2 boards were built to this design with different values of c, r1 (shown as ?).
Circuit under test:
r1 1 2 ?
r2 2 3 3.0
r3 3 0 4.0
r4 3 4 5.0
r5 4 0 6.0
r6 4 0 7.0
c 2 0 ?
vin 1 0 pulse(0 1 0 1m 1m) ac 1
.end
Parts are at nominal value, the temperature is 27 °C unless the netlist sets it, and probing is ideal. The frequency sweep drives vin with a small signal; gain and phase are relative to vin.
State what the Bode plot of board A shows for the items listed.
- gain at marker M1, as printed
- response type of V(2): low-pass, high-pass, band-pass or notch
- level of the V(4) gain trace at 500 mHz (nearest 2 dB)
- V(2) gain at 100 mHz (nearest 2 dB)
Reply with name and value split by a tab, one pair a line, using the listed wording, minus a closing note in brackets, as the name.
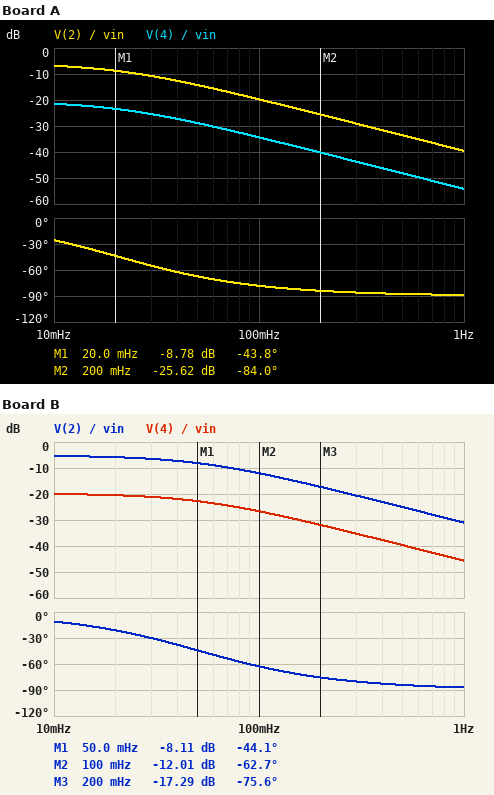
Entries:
gain at marker M1, as printed	-8.78 dB
response type of V(2): low-pass, high-pass, band-pass or notch	low-pass
level of the V(4) gain trace at 500 mHz	-48 dB
V(2) gain at 100 mHz	-20 dB
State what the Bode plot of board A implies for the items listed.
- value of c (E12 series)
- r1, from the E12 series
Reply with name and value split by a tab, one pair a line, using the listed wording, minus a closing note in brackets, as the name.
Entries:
value of c	2.7 F
r1, from the E12 series	5.6 Ω
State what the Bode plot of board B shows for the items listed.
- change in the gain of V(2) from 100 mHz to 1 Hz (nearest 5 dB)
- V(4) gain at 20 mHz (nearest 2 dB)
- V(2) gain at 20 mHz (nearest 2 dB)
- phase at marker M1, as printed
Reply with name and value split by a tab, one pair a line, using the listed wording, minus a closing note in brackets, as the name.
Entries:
change in the gain of V(2) from 100 mHz to 1 Hz	-20 dB
V(4) gain at 20 mHz	-20 dB
V(2) gain at 20 mHz	-6 dB
phase at marker M1, as printed	-44.1 deg
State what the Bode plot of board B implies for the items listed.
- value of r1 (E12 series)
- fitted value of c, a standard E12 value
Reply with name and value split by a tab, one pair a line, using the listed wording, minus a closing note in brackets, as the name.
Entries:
value of r1	4.7 Ω
fitted value of c, a standard E12 value	1.2 F
